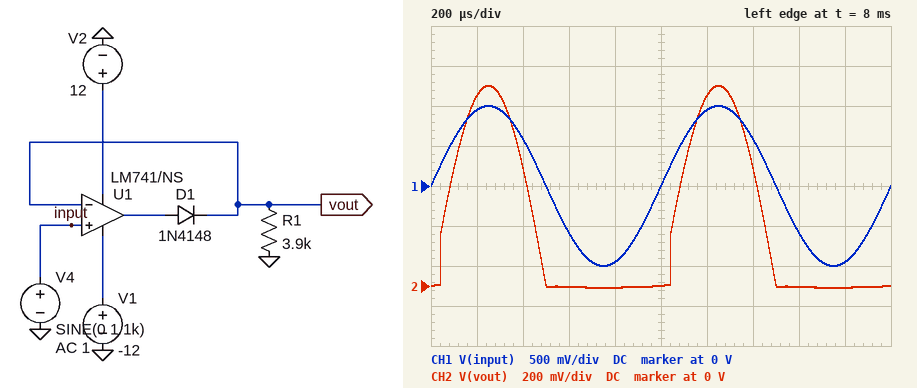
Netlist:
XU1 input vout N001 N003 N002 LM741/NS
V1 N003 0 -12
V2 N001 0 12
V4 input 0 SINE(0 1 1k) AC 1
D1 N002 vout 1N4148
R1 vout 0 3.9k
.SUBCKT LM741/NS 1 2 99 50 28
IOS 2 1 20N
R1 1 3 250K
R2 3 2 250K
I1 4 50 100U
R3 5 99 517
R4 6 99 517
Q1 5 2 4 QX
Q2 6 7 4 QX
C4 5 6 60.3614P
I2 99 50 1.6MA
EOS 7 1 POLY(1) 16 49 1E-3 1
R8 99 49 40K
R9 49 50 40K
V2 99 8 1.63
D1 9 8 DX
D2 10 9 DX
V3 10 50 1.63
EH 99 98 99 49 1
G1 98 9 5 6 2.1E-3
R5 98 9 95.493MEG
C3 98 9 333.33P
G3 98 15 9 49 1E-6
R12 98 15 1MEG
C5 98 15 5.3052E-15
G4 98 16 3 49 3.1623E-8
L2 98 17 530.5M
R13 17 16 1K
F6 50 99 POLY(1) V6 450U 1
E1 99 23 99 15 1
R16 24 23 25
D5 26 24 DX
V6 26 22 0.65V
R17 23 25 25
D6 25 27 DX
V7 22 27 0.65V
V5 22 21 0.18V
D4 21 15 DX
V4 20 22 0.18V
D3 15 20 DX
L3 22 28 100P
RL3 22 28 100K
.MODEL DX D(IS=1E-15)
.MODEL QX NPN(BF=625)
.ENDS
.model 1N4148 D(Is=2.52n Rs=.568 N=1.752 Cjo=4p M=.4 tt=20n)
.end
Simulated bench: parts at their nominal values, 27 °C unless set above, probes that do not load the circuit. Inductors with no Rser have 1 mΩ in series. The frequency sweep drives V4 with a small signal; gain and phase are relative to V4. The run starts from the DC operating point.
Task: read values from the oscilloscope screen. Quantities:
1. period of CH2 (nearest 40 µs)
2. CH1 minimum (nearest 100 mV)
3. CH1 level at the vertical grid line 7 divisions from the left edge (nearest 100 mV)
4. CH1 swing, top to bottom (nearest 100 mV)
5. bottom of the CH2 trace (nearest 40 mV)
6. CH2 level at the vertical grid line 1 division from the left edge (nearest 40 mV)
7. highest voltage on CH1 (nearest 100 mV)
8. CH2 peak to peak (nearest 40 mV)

1.00 ms
-1.0 V
600 mV
2.0 V
0 V
960 mV
1.0 V
1.00 V
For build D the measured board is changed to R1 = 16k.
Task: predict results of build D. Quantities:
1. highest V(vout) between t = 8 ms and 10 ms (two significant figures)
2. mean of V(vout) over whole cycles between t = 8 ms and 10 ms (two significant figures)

1.0 V
300 mV
